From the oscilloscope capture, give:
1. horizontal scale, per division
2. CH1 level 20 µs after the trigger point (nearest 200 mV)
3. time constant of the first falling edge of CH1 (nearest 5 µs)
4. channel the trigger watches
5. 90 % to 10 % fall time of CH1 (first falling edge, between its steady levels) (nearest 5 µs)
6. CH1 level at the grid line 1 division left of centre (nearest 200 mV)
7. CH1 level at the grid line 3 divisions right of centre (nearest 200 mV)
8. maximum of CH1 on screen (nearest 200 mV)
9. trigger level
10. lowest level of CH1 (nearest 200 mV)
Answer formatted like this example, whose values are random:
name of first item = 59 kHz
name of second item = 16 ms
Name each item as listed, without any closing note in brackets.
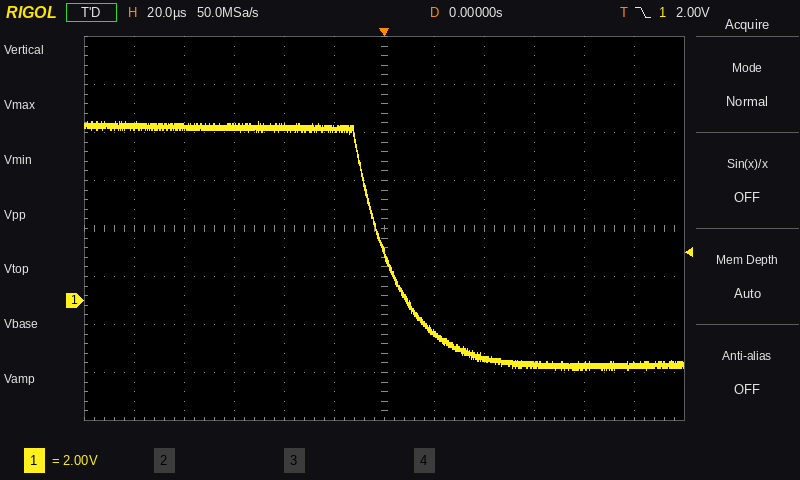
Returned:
horizontal scale, per division = 20 µs
CH1 level 20 µs after the trigger point = -1.4 V
time constant of the first falling edge of CH1 = 15 µs
channel the trigger watches = CH1
90 % to 10 % fall time of CH1 (first falling edge, between its steady levels) = 35 µs
CH1 level at the grid line 1 division left of centre = 7.2 V
CH1 level at the grid line 3 divisions right of centre = -2.6 V
maximum of CH1 on screen = 7.4 V
trigger level = 2.00 V
lowest level of CH1 = -2.8 V
